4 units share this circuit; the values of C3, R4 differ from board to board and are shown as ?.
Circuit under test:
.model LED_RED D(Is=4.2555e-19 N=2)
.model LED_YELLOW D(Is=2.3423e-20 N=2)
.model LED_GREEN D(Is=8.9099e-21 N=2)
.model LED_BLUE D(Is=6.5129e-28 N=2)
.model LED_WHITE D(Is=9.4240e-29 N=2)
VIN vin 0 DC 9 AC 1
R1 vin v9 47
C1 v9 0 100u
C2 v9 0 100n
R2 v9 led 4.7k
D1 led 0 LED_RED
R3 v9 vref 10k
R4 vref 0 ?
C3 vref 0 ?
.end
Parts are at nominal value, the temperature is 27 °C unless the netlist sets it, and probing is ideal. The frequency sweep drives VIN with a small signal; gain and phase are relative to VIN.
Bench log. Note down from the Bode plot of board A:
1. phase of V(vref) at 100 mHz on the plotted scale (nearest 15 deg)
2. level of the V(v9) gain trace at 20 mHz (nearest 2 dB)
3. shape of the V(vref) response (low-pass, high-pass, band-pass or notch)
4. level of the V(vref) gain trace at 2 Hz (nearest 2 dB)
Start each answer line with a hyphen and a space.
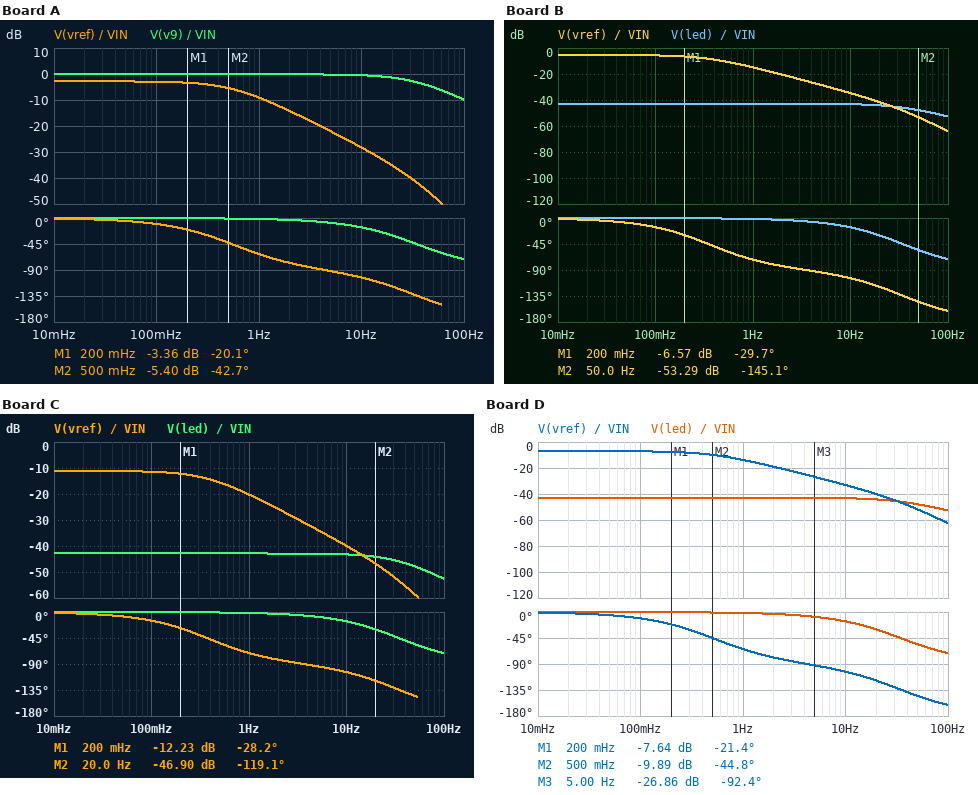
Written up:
- -15 deg
- 0 dB
- low-pass
- -14 dB
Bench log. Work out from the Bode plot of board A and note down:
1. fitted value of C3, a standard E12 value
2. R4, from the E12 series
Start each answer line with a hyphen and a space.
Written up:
- 39 µF
- 27 kΩ
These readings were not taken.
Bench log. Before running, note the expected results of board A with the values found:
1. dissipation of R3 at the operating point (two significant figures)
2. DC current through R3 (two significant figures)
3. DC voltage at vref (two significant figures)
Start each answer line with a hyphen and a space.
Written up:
- 580 µW
- 240 µA
- 6.5 V
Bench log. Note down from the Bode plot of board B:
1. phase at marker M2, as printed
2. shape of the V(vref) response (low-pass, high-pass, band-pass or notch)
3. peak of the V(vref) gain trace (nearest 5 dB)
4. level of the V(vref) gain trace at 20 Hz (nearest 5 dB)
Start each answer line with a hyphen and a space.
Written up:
- -145.1 deg
- low-pass
- -5 dB
- -40 dB
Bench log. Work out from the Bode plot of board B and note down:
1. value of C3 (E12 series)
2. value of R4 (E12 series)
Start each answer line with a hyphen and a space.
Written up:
- 82 µF
- 12 kΩ
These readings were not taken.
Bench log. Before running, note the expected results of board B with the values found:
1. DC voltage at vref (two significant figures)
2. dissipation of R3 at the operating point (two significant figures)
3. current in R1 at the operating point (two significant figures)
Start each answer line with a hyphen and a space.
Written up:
- 4.9 V
- 1.6 mW
- 1.9 mA
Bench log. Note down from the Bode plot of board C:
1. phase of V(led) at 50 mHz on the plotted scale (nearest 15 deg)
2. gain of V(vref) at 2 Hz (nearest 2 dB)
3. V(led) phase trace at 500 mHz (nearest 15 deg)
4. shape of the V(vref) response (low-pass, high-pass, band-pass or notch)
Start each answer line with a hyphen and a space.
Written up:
- 0 deg
- -26 dB
- 0 deg
- low-pass
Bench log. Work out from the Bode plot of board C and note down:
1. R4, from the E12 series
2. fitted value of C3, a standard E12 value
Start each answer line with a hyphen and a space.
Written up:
- 3.9 kΩ
- 150 µF
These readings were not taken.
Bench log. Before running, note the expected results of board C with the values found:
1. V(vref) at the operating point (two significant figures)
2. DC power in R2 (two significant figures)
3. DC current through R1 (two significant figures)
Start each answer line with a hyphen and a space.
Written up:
- 2.5 V
- 11 mW
- 2.1 mA
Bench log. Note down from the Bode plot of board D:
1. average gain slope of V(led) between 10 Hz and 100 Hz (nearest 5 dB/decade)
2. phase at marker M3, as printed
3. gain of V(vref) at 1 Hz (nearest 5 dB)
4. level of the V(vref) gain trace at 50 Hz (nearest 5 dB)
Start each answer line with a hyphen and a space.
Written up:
- -10 dB/decade
- -92.4 deg
- -15 dB
- -50 dB
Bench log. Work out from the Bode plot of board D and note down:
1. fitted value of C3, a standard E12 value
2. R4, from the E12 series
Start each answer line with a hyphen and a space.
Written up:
- 68 µF
- 8.2 kΩ
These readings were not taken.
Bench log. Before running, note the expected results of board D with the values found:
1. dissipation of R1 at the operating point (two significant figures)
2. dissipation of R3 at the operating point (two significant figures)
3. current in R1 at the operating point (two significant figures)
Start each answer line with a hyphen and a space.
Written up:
- 190 µW
- 2.4 mW
- 2.0 mA
